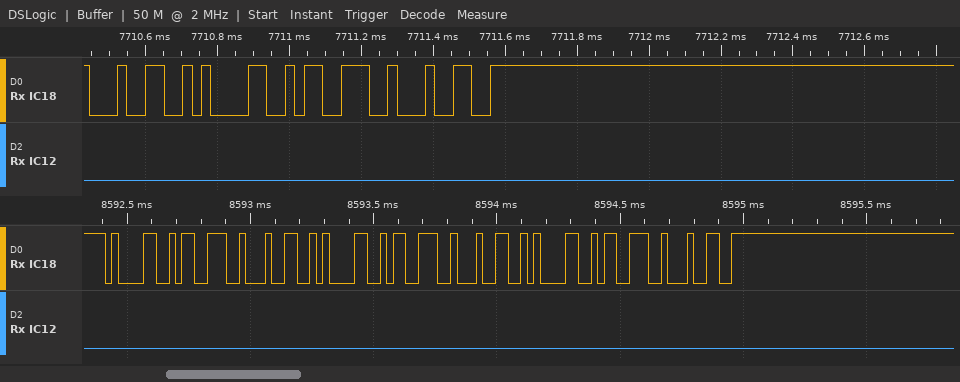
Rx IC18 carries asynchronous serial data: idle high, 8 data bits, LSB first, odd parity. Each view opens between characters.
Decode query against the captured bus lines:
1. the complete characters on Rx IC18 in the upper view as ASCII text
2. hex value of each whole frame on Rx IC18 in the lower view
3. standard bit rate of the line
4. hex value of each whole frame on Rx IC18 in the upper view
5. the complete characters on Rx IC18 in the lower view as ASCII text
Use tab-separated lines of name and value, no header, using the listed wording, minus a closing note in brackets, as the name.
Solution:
the complete characters on Rx IC18 in the upper view as ASCII text	"dasd"
hex value of each whole frame on Rx IC18 in the lower view	61, 73, 64, 61, 73, 64, 61, 73, 64
standard bit rate of the line	38400 baud
hex value of each whole frame on Rx IC18 in the upper view	64, 61, 73, 64
the complete characters on Rx IC18 in the lower view as ASCII text	"asdasdasd"
